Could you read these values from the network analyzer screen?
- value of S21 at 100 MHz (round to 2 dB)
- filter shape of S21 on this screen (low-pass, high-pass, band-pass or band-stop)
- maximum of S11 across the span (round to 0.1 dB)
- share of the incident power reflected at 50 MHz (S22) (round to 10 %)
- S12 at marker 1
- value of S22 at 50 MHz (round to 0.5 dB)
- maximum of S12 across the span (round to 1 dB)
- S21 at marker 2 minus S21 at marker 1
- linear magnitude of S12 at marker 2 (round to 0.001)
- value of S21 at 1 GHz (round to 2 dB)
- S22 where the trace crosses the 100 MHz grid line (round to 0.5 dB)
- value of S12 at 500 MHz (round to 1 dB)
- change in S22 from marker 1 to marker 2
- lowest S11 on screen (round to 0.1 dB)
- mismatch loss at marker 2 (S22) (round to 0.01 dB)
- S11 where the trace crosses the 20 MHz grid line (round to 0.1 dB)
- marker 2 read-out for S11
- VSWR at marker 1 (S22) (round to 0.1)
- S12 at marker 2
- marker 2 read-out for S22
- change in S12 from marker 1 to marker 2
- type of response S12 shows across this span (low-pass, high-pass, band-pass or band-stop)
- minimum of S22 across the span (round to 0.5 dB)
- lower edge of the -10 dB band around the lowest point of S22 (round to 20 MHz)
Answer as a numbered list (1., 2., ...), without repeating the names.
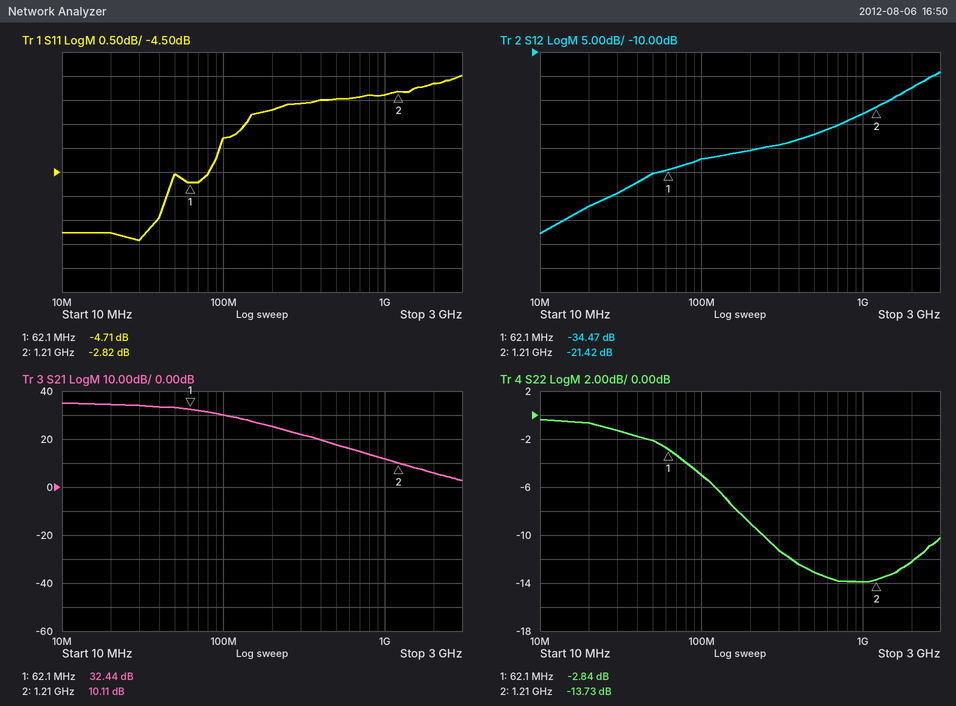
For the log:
1. 30 dB
2. low-pass
3. -2.5 dB
4. 60 %
5. -34.47 dB
6. -2.0 dB
7. -14 dB
8. -22.33 dB
9. 0.085
10. 12 dB
11. -5.0 dB
12. -27 dB
13. -10.89 dB
14. -5.9 dB
15. 0.19 dB
16. -5.8 dB
17. -2.82 dB
18. 6.2
19. -21.42 dB
20. -13.73 dB
21. 13.05 dB
22. high-pass
23. -14.0 dB
24. 240 MHz
